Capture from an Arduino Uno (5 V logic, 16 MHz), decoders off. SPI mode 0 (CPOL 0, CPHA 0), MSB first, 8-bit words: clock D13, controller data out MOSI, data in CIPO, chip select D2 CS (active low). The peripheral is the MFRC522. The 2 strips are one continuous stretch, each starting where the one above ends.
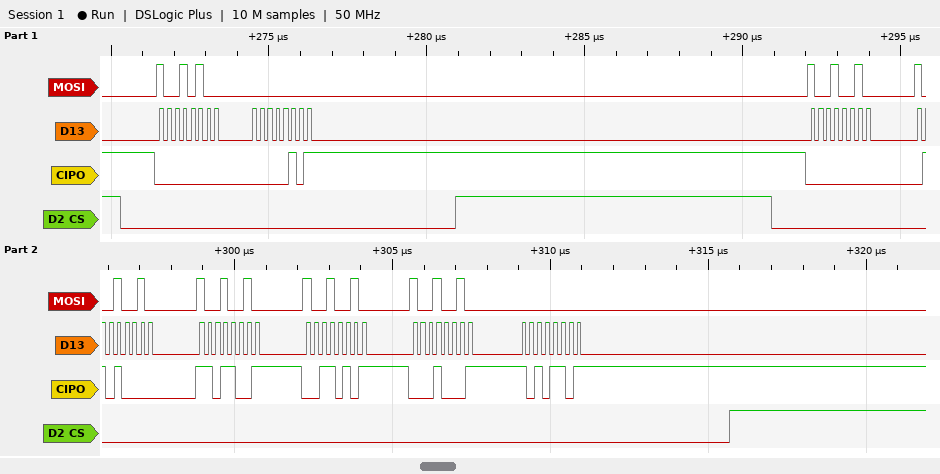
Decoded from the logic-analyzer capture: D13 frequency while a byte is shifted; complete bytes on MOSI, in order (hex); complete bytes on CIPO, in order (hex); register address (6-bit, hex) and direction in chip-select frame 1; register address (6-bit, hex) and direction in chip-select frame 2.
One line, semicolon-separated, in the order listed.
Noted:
4 MHz; 94 00 92 92 92 92 92 00; 00 05 00 50 D9 35 11 AD; 0x0A read; 0x09 read
